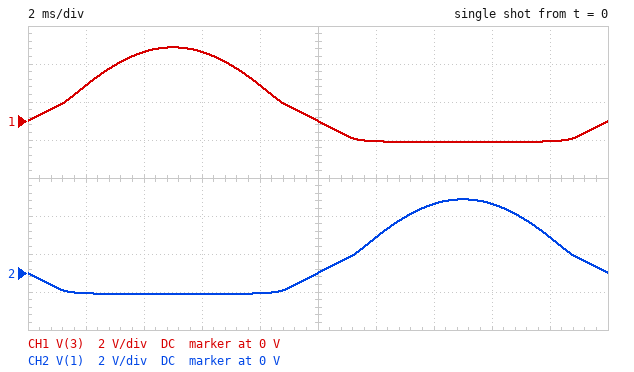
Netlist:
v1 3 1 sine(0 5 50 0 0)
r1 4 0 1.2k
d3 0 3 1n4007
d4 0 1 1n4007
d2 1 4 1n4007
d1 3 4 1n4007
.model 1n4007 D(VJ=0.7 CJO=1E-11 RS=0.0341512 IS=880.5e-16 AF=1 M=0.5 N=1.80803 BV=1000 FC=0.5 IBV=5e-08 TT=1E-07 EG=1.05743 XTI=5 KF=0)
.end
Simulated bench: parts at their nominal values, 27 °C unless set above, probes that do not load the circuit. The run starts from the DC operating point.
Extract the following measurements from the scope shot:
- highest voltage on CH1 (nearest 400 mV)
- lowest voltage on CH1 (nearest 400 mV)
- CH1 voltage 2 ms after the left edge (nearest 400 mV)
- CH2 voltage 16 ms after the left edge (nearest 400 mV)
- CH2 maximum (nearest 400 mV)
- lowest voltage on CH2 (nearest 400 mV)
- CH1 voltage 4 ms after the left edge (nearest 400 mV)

4.0 V
-1.2 V
2.0 V
3.6 V
4.0 V
-1.2 V
3.6 V
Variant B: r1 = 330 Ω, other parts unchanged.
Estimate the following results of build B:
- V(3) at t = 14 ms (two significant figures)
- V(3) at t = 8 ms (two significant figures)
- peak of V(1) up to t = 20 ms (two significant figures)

-1.2 V
1.8 V
3.8 V
